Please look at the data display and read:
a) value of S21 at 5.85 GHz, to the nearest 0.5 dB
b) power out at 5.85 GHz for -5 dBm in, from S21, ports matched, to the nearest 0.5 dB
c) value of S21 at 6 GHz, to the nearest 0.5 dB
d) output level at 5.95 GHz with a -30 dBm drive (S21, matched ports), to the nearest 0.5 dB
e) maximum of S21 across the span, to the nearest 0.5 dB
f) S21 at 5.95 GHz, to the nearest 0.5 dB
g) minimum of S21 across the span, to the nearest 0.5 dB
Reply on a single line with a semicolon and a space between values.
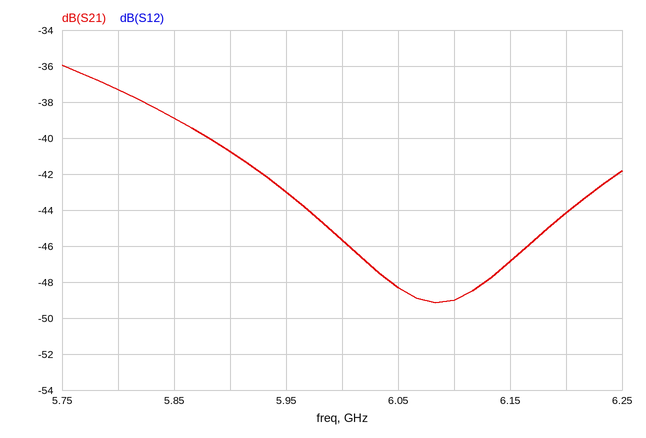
-39.0 dB; -44.0 dBm; -45.5 dB; -73.0 dBm; -36.0 dB; -43.0 dB; -49.0 dB
